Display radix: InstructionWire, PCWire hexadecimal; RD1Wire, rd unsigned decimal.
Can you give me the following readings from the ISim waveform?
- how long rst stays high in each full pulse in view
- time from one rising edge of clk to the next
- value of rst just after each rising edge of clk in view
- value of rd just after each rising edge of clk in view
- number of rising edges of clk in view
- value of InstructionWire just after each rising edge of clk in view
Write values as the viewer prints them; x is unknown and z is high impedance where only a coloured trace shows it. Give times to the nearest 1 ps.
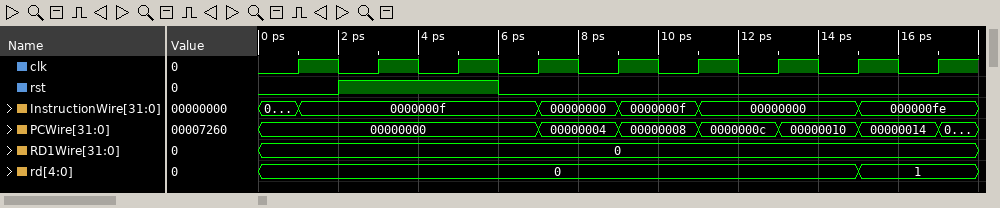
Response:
4 ps
2 ps
0 1 1 0 0 0 0 0 0
0, 0, 0, 0, 0, 0, 0, 1, 1
9
0000000f, 0000000f, 0000000f, 00000000, 0000000f, 00000000, 00000000, 000000fe, 000000fe
